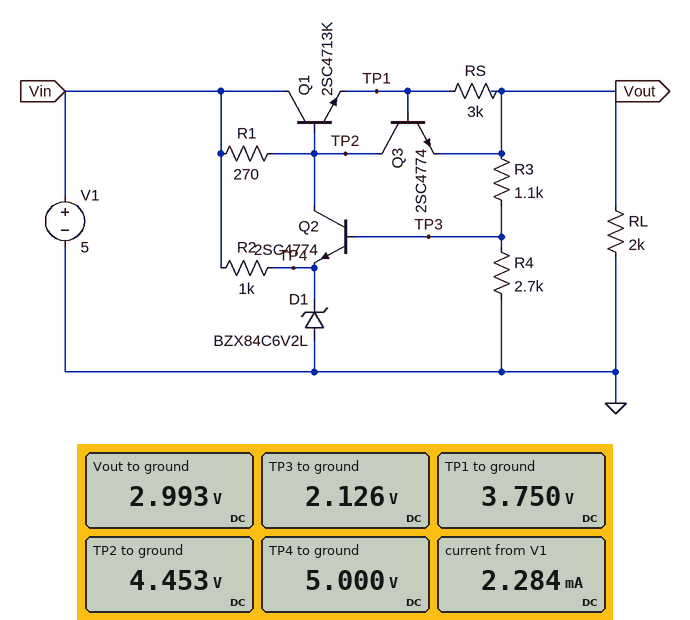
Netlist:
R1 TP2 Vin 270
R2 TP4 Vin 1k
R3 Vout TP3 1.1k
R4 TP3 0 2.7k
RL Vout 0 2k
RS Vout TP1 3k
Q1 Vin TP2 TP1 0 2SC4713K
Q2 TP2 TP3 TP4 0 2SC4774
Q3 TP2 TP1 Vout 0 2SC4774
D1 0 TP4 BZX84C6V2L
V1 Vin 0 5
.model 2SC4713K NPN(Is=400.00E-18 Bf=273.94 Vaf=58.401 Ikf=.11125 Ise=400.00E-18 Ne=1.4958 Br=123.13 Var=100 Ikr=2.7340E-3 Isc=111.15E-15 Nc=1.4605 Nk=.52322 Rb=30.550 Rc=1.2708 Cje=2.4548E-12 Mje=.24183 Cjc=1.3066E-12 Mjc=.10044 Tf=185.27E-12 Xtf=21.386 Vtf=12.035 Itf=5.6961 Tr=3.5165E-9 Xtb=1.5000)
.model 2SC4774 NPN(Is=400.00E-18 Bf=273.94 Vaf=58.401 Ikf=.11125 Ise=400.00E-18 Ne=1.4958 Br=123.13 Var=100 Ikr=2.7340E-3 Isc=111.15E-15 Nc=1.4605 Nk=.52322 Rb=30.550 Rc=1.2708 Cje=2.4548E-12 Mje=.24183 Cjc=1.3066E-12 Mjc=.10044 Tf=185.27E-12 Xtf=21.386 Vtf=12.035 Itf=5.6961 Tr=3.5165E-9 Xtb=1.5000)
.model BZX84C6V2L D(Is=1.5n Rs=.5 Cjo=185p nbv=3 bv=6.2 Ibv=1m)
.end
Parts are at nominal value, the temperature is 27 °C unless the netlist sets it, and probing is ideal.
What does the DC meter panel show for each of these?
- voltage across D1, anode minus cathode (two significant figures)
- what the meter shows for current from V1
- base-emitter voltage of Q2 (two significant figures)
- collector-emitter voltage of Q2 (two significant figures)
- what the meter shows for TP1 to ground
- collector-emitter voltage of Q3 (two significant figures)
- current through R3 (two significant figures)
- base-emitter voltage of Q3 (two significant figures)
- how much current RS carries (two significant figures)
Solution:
-5.0 V
2.284 mA
-2.9 V
-550 mV
3.750 V
1.5 V
790 µA
760 mV
250 µA
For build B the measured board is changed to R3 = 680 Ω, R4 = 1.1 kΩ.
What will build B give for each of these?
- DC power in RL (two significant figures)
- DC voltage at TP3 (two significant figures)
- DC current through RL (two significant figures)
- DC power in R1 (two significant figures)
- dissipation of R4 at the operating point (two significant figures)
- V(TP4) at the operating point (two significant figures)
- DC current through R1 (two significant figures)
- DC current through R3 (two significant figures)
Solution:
3.9 mW
1.7 V
1.4 mA
2.0 mW
2.7 mW
5.0 V
2.7 mA
1.6 mA
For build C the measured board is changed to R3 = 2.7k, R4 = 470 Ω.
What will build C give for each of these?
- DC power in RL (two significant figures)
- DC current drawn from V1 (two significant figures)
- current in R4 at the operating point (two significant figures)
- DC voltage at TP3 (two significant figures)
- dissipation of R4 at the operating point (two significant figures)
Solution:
4.4 mW
2.4 mA
930 µA
440 mV
410 µW
